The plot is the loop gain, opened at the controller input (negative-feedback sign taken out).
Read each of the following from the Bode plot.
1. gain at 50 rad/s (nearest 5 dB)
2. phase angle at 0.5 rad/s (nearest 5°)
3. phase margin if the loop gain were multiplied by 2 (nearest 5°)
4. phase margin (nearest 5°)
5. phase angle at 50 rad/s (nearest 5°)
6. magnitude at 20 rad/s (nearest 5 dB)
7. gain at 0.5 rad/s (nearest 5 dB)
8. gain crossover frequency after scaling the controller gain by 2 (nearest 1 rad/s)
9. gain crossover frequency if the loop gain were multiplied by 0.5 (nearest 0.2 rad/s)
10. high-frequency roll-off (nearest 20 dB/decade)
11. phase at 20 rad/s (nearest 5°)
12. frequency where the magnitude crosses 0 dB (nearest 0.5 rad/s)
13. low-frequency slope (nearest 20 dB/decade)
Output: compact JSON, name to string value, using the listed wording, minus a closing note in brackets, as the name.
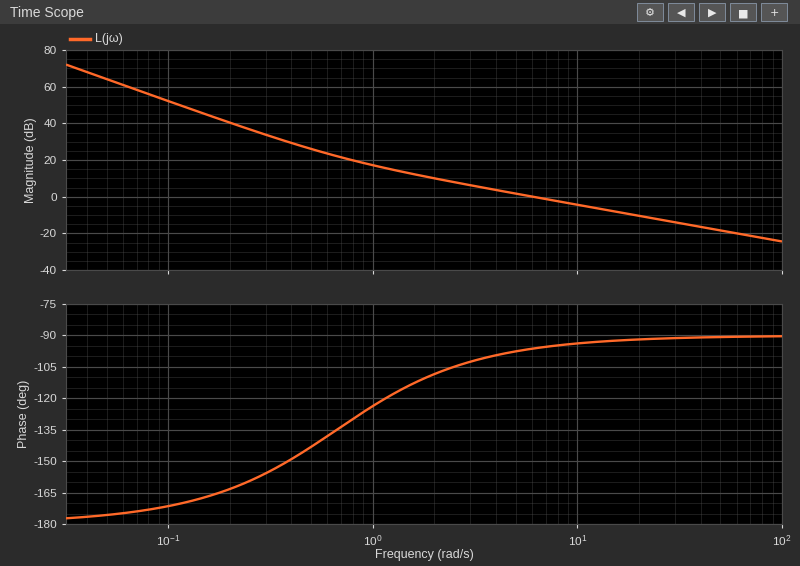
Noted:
{"gain at 50 rad/s": "-20 dB", "phase angle at 0.5 rad/s": "-145°", "phase margin if the loop gain were multiplied by 2": "85°", "phase margin": "85°", "phase angle at 50 rad/s": "-90°", "magnitude at 20 rad/s": "-10 dB", "gain at 0.5 rad/s": "25 dB", "gain crossover frequency after scaling the controller gain by 2": "12 rad/s", "gain crossover frequency if the loop gain were multiplied by 0.5": "3.0 rad/s", "high-frequency roll-off": "-20 dB/decade", "phase at 20 rad/s": "-90°", "frequency where the magnitude crosses 0 dB": "6.0 rad/s", "low-frequency slope": "-40 dB/decade"}
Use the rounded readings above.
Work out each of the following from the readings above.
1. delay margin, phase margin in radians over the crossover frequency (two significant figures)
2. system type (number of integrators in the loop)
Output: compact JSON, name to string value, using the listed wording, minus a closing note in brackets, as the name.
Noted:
{"delay margin, phase margin in radians over the crossover frequency": "0.25 s", "system type": "2"}
